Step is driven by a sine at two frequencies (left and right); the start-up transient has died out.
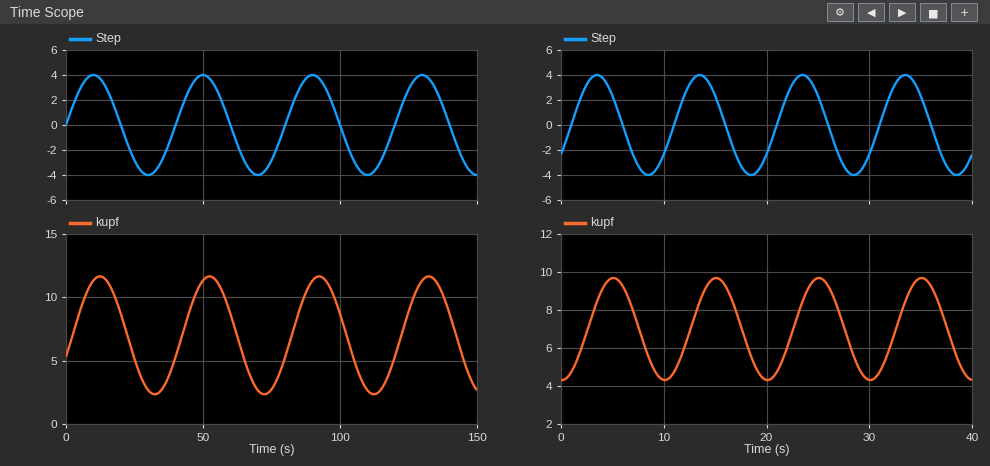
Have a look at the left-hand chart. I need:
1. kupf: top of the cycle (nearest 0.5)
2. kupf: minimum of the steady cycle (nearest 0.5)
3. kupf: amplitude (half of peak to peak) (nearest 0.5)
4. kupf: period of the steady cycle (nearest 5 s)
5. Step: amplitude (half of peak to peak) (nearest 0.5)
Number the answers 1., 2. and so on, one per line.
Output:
1. 11.5
2. 2.5
3. 4.5
4. 40 s
5. 4.0
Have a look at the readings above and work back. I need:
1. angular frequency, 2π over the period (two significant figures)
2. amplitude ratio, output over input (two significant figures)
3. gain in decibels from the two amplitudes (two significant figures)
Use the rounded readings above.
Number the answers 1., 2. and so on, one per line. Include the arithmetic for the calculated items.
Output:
1. 2π / 40 = 0.16 rad/s
2. 4.5 / 4 = 1.1
3. 20 log10(4.5 / 4) = 1.0 dB
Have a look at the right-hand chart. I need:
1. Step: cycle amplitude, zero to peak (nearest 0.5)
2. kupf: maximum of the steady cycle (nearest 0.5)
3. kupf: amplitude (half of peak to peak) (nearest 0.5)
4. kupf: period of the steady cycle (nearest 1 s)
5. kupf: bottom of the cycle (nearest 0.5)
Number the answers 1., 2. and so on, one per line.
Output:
1. 4.0
2. 9.5
3. 2.5
4. 10 s
5. 4.5
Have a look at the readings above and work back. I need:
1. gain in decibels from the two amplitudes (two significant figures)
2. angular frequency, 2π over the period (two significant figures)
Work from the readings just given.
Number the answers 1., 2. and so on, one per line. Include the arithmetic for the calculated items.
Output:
1. 20 log10(2.5 / 4) = -4.1 dB
2. 2π / 10 = 0.63 rad/s
